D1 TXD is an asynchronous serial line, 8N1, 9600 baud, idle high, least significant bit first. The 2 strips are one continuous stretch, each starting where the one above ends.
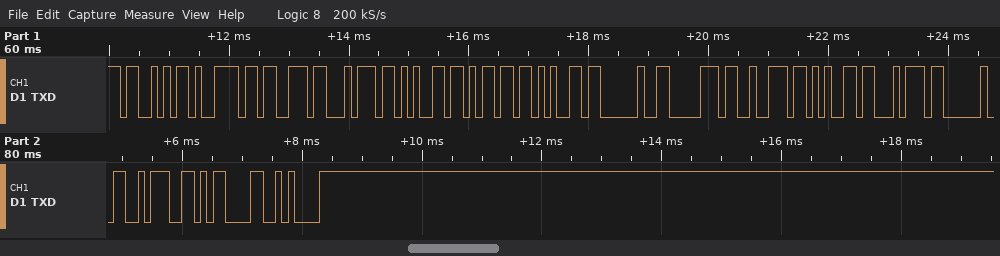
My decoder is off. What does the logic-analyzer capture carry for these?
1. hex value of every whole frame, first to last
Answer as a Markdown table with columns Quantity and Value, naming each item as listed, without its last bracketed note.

| Quantity | Value |
|---|---|
| hex value of every whole frame, first to last | 0x53 0x79 0x73 0x74 0x65 0x6D 0x65 0x20 0x70 0x72 0x65 0x74 0x20 0x3A 0x0D 0x0A |
